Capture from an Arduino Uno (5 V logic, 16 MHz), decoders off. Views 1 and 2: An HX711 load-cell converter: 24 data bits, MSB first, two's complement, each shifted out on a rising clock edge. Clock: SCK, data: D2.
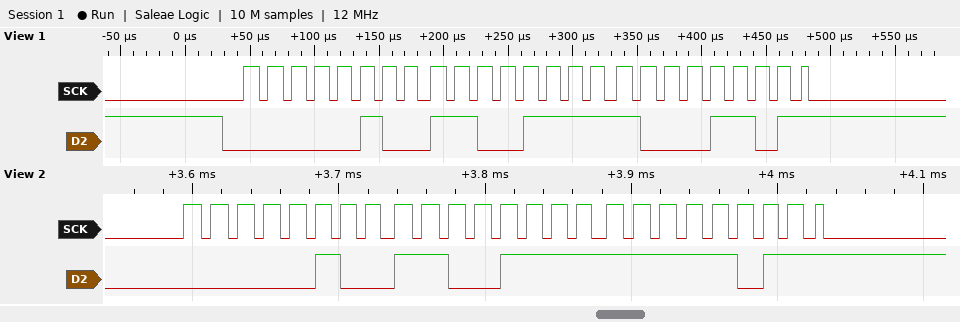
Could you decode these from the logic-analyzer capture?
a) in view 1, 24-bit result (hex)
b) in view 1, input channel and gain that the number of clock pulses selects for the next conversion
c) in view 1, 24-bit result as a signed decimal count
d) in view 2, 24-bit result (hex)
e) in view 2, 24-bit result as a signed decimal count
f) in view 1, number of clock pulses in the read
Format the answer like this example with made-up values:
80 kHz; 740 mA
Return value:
0x04CF8D; channel A, gain 128; 315277; 0x04CFFB; 315387; 25
